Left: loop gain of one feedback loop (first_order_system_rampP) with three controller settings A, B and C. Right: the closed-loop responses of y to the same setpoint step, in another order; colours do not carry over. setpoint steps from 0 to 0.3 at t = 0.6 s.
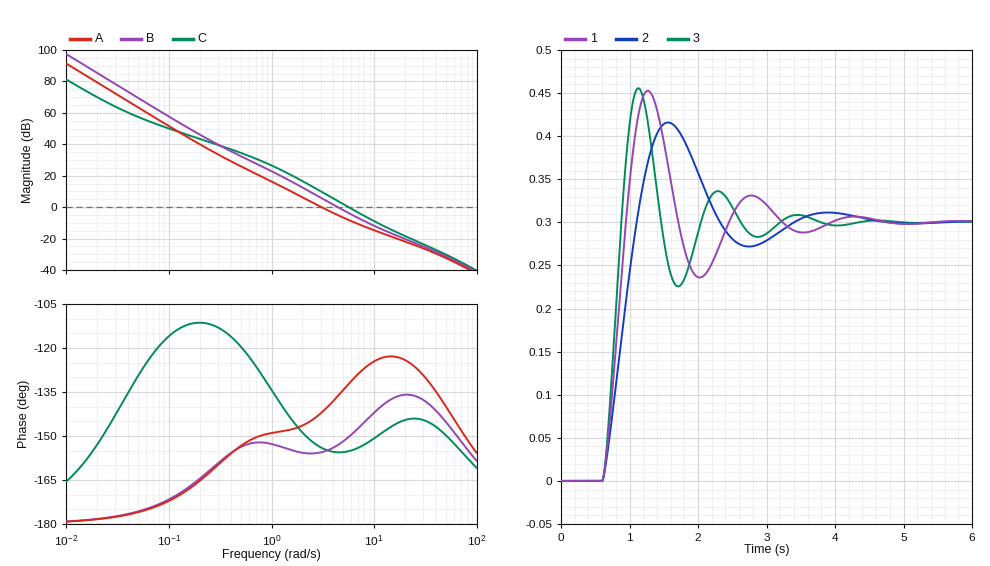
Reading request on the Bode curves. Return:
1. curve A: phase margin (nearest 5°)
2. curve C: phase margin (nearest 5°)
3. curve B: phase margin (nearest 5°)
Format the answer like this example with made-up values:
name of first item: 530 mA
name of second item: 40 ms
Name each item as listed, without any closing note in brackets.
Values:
curve A: phase margin: 40°
curve C: phase margin: 25°
curve B: phase margin: 25°
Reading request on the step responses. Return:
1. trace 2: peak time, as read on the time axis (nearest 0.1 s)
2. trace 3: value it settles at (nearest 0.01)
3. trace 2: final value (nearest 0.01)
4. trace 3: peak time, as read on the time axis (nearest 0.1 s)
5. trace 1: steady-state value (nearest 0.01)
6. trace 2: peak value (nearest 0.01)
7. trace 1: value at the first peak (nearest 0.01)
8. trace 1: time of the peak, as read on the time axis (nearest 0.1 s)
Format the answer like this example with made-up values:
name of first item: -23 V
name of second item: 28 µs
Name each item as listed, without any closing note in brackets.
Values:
trace 2: peak time, as read on the time axis: 1.6 s
trace 3: value it settles at: 0.30
trace 2: final value: 0.30
trace 3: peak time, as read on the time axis: 1.1 s
trace 1: steady-state value: 0.30
trace 2: peak value: 0.42
trace 1: value at the first peak: 0.45
trace 1: time of the peak, as read on the time axis: 1.3 s
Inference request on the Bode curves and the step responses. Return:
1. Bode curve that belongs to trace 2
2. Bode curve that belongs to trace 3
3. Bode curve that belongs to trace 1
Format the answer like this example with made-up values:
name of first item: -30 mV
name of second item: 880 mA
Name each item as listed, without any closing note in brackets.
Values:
Bode curve that belongs to trace 2: A
Bode curve that belongs to trace 3: C
Bode curve that belongs to trace 1: B
